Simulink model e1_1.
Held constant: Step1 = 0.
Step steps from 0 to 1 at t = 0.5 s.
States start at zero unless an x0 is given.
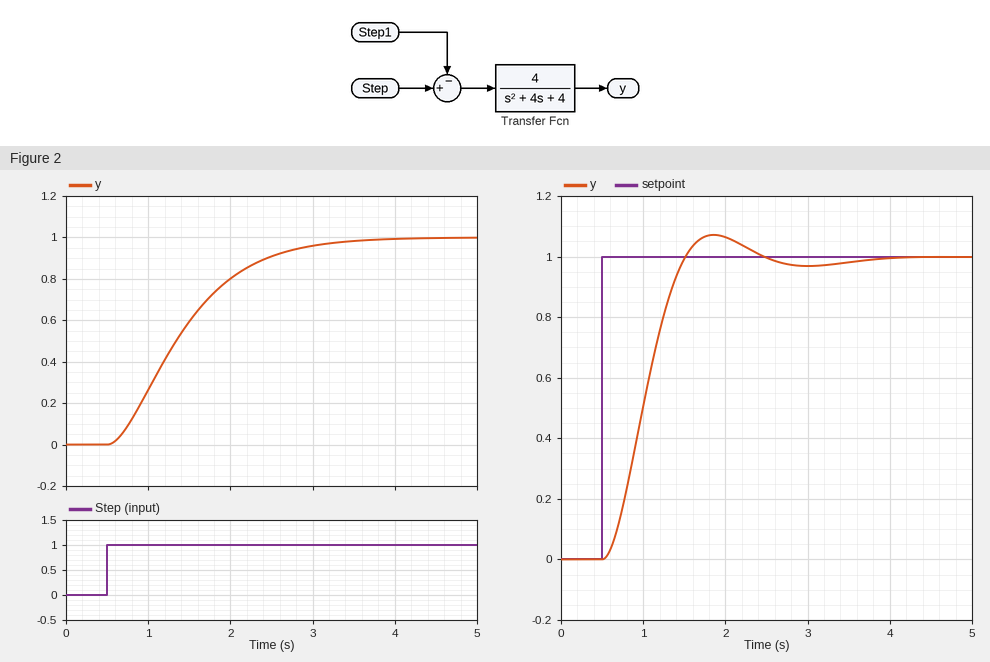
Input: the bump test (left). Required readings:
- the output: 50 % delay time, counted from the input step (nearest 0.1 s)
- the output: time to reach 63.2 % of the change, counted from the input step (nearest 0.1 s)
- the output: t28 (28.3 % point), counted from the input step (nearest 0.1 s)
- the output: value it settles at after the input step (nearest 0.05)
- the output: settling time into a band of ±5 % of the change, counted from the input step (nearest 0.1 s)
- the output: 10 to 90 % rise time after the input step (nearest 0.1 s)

0.8 s
1.1 s
0.5 s
1.00
2.4 s
1.7 s
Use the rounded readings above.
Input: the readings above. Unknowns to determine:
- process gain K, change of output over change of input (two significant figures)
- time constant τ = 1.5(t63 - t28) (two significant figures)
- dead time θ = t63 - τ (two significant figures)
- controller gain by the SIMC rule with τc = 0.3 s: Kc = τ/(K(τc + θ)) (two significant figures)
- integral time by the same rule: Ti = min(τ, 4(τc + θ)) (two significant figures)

1.0
0.90 s
0.20 s
1.8
0.90 s
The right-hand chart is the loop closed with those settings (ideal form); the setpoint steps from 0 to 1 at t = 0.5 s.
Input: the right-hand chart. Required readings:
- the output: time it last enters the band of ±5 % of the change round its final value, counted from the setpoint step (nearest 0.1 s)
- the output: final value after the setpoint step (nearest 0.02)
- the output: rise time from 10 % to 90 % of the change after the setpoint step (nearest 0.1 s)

1.6 s
1.00
0.7 s
